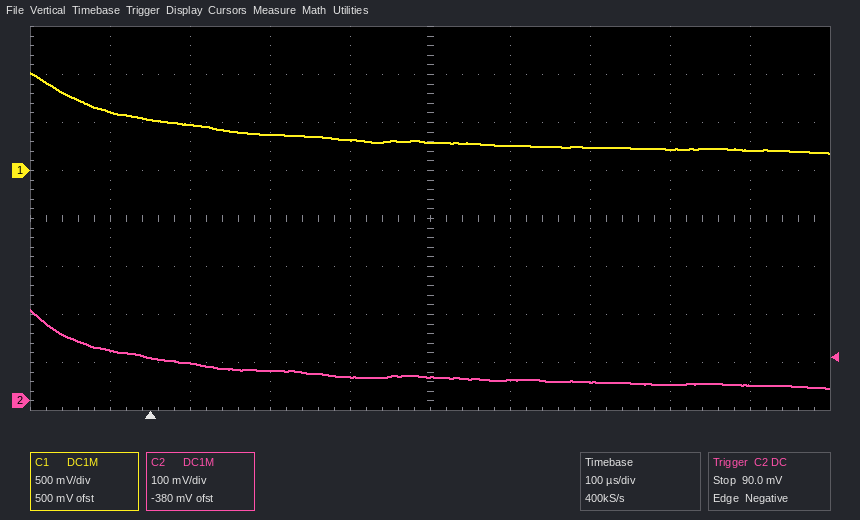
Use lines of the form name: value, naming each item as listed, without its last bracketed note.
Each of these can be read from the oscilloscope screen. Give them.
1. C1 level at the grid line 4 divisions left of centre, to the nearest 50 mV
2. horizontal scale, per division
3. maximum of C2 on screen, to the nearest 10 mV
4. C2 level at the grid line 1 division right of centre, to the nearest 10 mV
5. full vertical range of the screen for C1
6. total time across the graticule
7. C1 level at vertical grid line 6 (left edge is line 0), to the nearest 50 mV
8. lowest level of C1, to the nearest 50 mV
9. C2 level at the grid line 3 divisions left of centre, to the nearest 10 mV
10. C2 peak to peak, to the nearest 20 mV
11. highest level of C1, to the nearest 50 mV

C1 level at the grid line 4 divisions left of centre, to the nearest 50 mV: 600 mV
horizontal scale, per division: 100 µs
maximum of C2 on screen, to the nearest 10 mV: 190 mV
C2 level at the grid line 1 division right of centre, to the nearest 10 mV: 40 mV
full vertical range of the screen for C1: 4 V
total time across the graticule: 1 ms
C1 level at vertical grid line 6 (left edge is line 0), to the nearest 50 mV: 250 mV
lowest level of C1, to the nearest 50 mV: 200 mV
C2 level at the grid line 3 divisions left of centre, to the nearest 10 mV: 80 mV
C2 peak to peak, to the nearest 20 mV: 160 mV
highest level of C1, to the nearest 50 mV: 1.00 V
